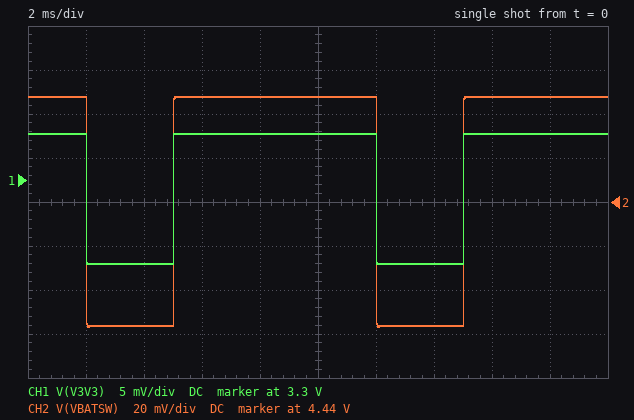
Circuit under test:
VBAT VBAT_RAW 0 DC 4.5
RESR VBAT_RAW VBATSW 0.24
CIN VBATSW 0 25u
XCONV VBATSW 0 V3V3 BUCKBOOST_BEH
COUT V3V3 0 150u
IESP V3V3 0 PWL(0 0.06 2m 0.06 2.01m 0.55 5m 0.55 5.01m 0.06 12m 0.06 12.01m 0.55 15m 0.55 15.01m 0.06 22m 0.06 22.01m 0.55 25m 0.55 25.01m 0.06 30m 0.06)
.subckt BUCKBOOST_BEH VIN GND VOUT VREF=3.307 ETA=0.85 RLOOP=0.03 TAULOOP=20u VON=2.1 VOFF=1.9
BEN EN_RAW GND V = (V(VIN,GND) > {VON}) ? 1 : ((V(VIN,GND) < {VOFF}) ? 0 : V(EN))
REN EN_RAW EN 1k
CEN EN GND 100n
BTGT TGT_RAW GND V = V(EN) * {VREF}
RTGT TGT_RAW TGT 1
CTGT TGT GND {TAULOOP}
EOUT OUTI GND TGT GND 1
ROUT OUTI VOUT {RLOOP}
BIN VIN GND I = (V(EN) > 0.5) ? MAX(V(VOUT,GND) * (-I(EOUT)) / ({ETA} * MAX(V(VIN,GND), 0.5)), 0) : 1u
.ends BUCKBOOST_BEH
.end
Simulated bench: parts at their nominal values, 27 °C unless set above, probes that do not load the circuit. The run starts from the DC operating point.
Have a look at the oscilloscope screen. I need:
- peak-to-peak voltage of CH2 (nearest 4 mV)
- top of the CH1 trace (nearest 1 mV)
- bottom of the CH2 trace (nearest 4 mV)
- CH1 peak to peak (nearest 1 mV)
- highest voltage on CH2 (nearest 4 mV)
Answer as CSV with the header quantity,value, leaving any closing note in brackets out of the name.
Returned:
quantity,value
peak-to-peak voltage of CH2,104 mV
top of the CH1 trace,3.305 V
bottom of the CH2 trace,4.384 V
CH1 peak to peak,15 mV
highest voltage on CH2,4.488 V
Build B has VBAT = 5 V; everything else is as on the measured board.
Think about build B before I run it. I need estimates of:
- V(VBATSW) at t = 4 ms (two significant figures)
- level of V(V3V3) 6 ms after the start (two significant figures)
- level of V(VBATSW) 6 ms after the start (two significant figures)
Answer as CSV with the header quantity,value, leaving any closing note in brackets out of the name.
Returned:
quantity,value
V(VBATSW) at t = 4 ms,4.9 V
level of V(V3V3) 6 ms after the start,3.3 V
level of V(VBATSW) 6 ms after the start,5.0 V
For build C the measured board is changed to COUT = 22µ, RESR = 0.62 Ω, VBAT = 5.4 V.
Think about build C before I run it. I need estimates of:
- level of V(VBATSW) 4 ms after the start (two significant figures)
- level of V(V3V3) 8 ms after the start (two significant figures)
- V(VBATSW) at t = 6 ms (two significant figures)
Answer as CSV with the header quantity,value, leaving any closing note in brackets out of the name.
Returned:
quantity,value
level of V(VBATSW) 4 ms after the start,5.1 V
level of V(V3V3) 8 ms after the start,3.3 V
V(VBATSW) at t = 6 ms,5.4 V
